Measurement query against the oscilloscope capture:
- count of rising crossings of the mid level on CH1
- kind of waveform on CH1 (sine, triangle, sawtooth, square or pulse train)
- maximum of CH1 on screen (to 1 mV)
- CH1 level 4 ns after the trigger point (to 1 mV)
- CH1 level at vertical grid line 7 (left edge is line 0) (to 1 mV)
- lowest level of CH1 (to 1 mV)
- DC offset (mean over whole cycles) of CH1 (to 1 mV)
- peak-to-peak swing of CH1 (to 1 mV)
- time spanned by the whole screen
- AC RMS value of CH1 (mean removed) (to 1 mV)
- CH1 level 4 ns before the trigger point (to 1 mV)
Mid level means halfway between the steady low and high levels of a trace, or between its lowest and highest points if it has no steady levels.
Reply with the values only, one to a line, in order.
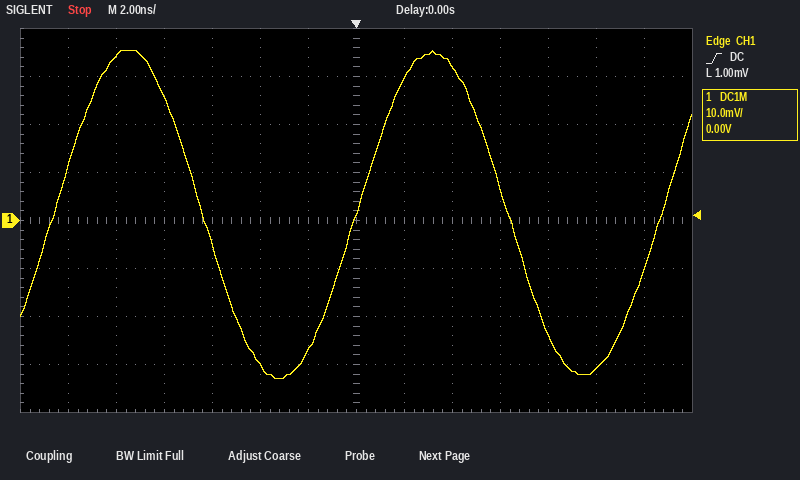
3
sine
35 mV
32 mV
1 mV
-33 mV
1 mV
68 mV
28 ns
24 mV
-30 mV
